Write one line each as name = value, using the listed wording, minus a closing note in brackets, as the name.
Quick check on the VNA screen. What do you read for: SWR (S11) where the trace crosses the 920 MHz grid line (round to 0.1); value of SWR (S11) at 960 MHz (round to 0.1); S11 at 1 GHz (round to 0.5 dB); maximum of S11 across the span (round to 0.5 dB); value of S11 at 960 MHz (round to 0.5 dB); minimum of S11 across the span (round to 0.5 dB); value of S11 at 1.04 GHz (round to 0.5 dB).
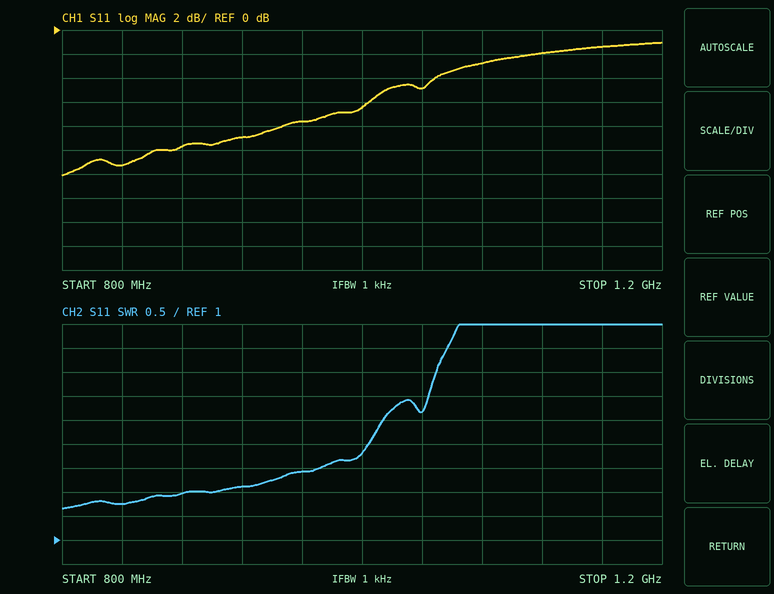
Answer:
SWR (S11) where the trace crosses the 920 MHz grid line = 2.1
value of SWR (S11) at 960 MHz = 2.4
S11 at 1 GHz = -6.5 dB
maximum of S11 across the span = -1.0 dB
value of S11 at 960 MHz = -7.5 dB
minimum of S11 across the span = -12.0 dB
value of S11 at 1.04 GHz = -5.0 dB
